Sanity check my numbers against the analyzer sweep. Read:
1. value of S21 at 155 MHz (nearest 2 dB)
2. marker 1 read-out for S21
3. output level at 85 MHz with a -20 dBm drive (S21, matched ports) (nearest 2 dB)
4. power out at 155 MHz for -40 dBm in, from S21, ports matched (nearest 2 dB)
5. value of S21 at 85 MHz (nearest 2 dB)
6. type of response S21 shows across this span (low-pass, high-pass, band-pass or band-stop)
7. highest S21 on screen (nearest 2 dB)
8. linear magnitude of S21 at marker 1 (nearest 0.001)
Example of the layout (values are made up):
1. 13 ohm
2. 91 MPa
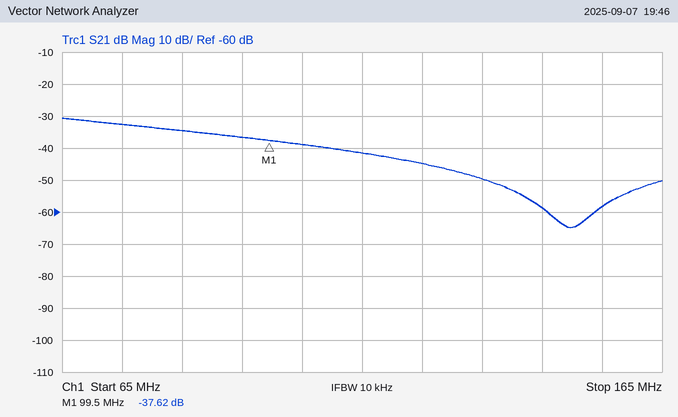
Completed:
1. -58 dB
2. -37.62 dB
3. -54 dBm
4. -98 dBm
5. -34 dB
6. low-pass
7. -30 dB
8. 0.013
